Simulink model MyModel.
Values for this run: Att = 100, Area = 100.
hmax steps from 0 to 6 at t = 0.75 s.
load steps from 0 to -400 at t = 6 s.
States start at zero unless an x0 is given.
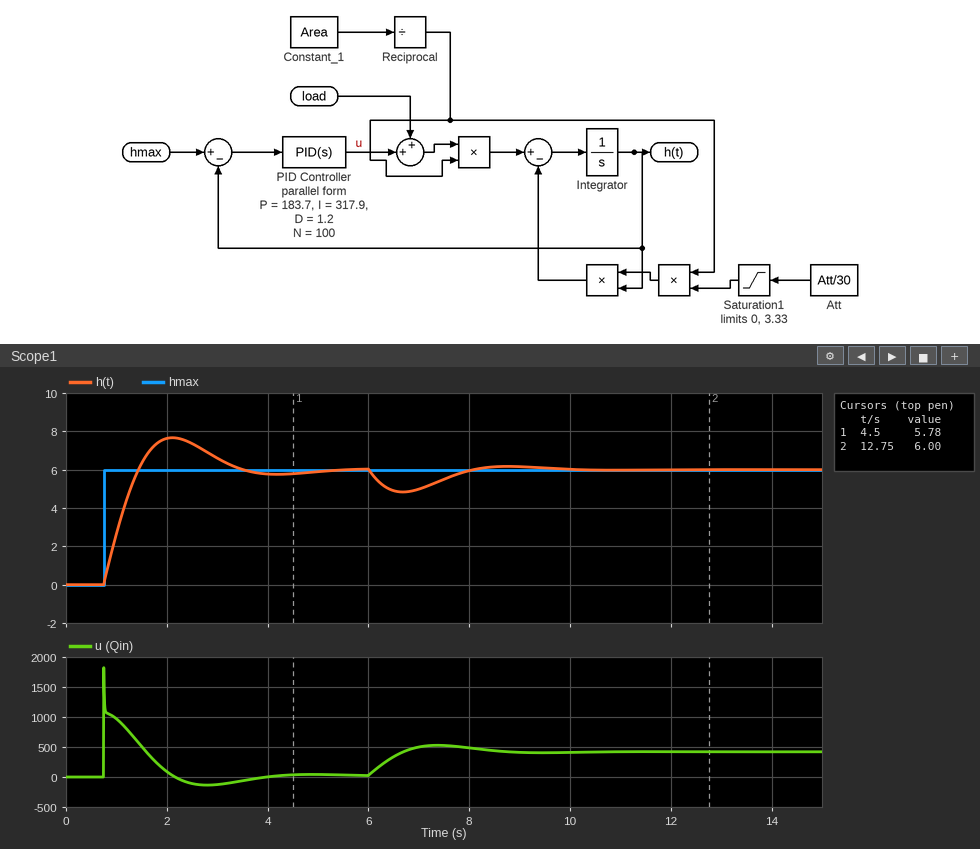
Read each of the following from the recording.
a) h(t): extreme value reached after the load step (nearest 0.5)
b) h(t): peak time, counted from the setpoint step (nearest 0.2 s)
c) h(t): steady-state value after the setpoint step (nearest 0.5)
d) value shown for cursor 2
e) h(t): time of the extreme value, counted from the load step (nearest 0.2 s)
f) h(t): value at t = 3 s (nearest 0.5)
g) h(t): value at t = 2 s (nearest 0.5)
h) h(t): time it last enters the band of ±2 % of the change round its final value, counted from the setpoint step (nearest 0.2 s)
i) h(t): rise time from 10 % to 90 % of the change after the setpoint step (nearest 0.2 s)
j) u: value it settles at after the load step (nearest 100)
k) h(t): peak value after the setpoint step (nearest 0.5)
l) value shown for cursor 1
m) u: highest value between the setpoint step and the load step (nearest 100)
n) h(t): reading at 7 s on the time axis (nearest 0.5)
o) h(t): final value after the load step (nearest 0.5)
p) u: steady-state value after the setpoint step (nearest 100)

5.0
1.4 s
6.0
6.00
0.6 s
6.5
7.5
4.2 s
0.6 s
400
7.5
5.78
1800
5.0
6.0
0
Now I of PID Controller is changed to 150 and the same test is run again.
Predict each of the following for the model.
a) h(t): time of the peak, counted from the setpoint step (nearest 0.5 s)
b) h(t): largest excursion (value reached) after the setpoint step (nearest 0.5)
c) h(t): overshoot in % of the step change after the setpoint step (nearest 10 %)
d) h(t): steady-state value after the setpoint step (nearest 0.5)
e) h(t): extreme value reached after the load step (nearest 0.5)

2.0 s
7.0
20 %
6.0
4.5
